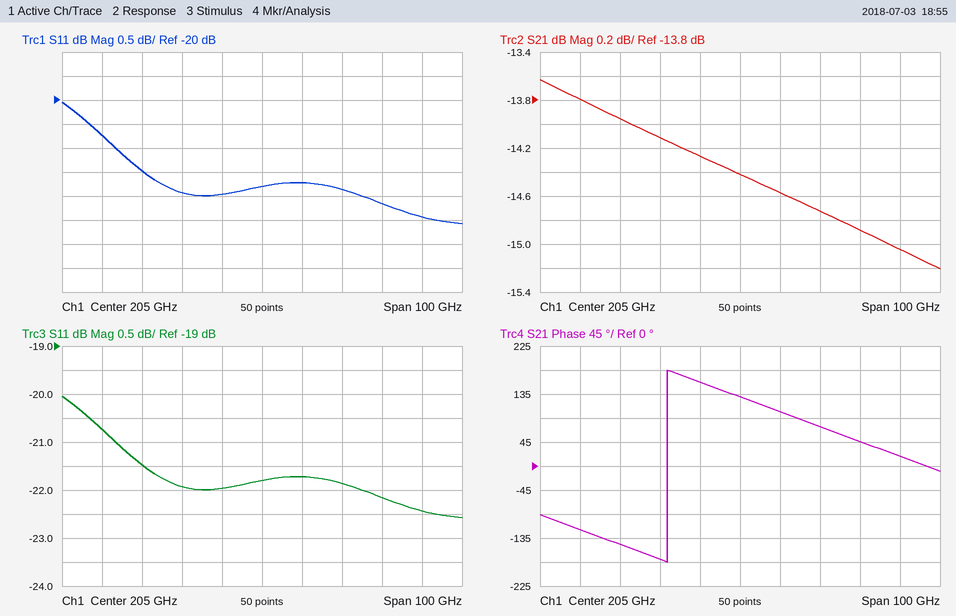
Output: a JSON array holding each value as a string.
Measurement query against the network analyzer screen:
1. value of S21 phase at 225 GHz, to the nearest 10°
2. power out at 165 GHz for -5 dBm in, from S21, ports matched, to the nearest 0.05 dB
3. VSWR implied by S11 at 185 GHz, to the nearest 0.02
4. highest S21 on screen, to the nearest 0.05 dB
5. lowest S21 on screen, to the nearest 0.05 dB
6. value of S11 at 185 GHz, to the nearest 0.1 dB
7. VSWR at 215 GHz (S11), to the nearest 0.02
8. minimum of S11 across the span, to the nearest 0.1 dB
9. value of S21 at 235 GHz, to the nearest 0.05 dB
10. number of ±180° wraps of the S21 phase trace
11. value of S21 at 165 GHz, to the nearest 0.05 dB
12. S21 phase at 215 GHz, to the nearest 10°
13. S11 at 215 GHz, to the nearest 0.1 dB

["70°", "-18.80 dBm", "1.18", "-13.65 dB", "-15.20 dB", "-21.9 dB", "1.18", "-22.6 dB", "-14.90 dB", "1", "-13.80 dB", "100°", "-21.7 dB"]
